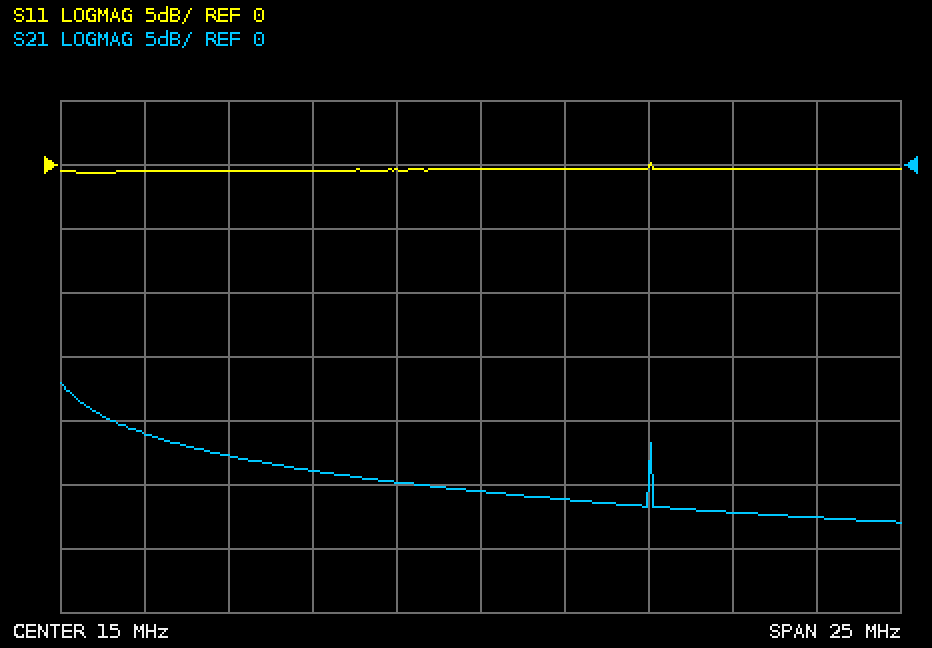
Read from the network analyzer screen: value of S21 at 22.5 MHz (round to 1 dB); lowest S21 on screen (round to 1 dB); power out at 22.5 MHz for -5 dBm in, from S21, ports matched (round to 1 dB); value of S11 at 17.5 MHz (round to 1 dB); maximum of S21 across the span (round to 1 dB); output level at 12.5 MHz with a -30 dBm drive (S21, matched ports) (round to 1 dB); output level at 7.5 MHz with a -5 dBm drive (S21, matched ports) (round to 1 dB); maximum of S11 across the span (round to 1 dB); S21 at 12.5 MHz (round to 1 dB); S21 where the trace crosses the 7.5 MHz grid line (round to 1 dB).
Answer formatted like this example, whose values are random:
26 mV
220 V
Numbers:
-27 dB
-28 dB
-32 dBm
0 dB
-17 dB
-55 dBm
-28 dBm
0 dB
-25 dB
-23 dB
